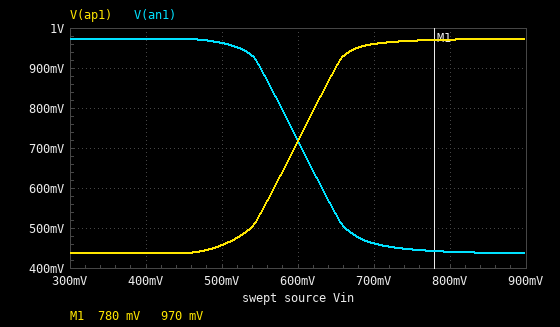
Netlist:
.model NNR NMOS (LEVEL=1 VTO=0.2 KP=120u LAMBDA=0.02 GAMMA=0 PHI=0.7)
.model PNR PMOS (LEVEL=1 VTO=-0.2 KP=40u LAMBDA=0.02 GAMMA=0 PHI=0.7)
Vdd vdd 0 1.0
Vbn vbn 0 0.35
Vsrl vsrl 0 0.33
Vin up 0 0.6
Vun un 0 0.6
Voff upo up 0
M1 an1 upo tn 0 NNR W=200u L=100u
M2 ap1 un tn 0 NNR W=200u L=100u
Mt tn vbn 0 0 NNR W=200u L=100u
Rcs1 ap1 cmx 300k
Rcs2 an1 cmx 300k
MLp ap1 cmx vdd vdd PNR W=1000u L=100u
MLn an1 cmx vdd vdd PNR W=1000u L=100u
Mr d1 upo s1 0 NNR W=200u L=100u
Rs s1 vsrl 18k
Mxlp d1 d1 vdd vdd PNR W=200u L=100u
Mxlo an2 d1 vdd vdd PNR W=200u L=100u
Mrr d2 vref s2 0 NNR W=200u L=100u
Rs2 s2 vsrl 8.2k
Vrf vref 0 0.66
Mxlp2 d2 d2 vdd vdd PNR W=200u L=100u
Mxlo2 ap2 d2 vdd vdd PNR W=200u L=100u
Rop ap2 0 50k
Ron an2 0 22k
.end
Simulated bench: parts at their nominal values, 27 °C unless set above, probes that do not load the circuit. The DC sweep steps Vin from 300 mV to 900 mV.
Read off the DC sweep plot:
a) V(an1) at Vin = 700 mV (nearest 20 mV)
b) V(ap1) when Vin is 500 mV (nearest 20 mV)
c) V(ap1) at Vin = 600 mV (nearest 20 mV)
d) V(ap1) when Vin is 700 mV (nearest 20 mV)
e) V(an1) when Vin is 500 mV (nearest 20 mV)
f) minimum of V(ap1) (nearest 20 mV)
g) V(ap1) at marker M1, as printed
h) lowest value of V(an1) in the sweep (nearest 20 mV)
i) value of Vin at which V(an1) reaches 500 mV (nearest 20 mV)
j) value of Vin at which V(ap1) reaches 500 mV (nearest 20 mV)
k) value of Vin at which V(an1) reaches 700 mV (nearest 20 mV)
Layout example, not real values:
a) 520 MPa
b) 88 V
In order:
a) 460 mV
b) 460 mV
c) 720 mV
d) 960 mV
e) 960 mV
f) 440 mV
g) 970 mV
h) 440 mV
i) 660 mV
j) 540 mV
k) 600 mV
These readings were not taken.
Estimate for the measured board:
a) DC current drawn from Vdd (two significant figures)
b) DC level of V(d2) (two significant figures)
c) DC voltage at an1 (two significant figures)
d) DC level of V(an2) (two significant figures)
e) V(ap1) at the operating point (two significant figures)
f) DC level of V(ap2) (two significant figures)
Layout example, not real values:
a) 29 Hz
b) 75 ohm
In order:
a) 6.9 µA
b) 600 mV
c) 720 mV
d) 10 mV
e) 720 mV
f) 83 mV
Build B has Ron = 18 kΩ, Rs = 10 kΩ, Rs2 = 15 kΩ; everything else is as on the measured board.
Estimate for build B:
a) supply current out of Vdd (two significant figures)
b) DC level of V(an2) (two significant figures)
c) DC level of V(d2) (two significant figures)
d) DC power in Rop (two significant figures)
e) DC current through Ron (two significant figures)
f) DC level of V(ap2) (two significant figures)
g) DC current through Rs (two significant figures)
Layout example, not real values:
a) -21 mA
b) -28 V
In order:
a) 6.6 µA
b) 9.3 mV
c) 610 mV
d) 100 nW
e) 520 nA
f) 72 mV
g) 510 nA
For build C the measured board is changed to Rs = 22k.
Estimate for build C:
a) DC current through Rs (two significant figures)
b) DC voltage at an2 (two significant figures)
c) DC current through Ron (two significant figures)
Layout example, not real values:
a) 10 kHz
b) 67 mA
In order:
a) 440 nA
b) 9.8 mV
c) 450 nA
